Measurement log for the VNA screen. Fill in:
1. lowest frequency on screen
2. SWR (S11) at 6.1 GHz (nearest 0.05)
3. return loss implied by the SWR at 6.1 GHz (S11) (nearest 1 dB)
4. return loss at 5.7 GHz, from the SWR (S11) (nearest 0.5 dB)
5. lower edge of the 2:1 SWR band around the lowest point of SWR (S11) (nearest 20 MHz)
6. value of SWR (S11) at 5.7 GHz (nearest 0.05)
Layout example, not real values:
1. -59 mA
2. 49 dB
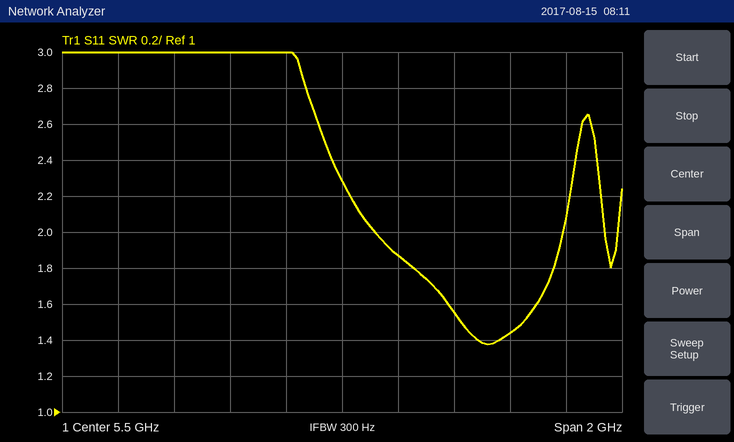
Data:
1. 4.5 GHz
2. 1.45
3. 15 dB
4. 10.5 dB
5. 5.62 GHz
6. 1.85
